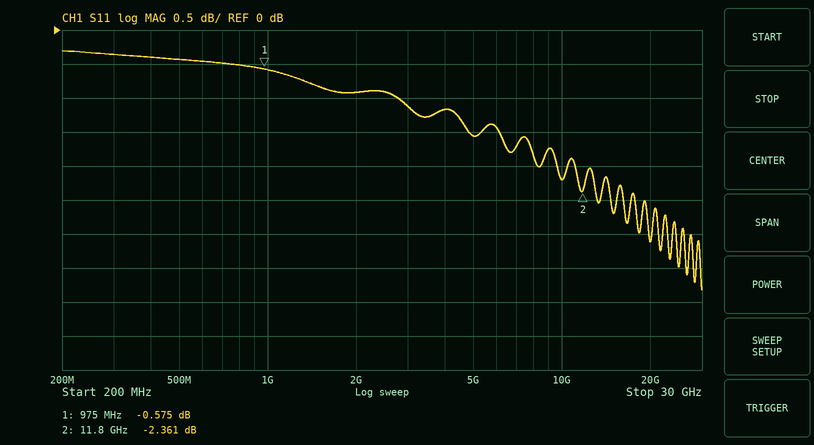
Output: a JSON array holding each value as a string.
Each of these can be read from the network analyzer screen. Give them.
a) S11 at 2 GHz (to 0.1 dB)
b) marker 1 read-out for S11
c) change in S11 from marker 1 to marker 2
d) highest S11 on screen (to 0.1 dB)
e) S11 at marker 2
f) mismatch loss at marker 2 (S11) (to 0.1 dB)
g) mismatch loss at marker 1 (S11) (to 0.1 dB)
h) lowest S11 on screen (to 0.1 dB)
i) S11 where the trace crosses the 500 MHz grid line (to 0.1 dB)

["-0.9 dB", "-0.575 dB", "-1.786 dB", "-0.3 dB", "-2.361 dB", "3.8 dB", "9.1 dB", "-3.8 dB", "-0.4 dB"]
